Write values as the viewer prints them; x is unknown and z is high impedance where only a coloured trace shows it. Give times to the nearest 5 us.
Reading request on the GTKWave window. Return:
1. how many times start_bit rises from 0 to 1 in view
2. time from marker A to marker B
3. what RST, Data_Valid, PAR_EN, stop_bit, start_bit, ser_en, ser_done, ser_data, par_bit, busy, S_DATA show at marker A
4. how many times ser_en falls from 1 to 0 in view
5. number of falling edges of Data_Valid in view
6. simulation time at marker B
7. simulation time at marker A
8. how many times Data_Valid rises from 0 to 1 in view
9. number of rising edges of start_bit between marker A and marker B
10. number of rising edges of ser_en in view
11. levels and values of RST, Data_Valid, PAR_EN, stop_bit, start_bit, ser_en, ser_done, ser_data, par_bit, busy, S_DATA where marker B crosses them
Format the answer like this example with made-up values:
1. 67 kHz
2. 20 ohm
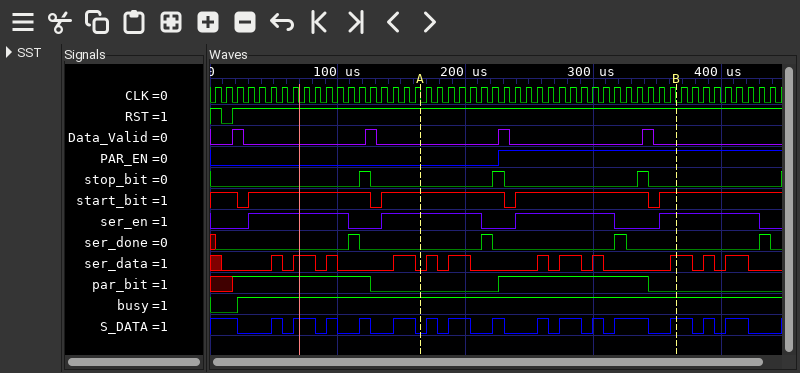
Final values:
1. 4
2. 200 us
3. RST=1, Data_Valid=0, PAR_EN=0, stop_bit=0, start_bit=1, ser_en=1, ser_done=0, ser_data=0, par_bit=0, busy=1, S_DATA=0
4. 4
5. 4
6. 365 us
7. 165 us
8. 4
9. 2
10. 4
11. RST=1, Data_Valid=0, PAR_EN=1, stop_bit=0, start_bit=1, ser_en=1, ser_done=0, ser_data=1, par_bit=0, busy=1, S_DATA=1
